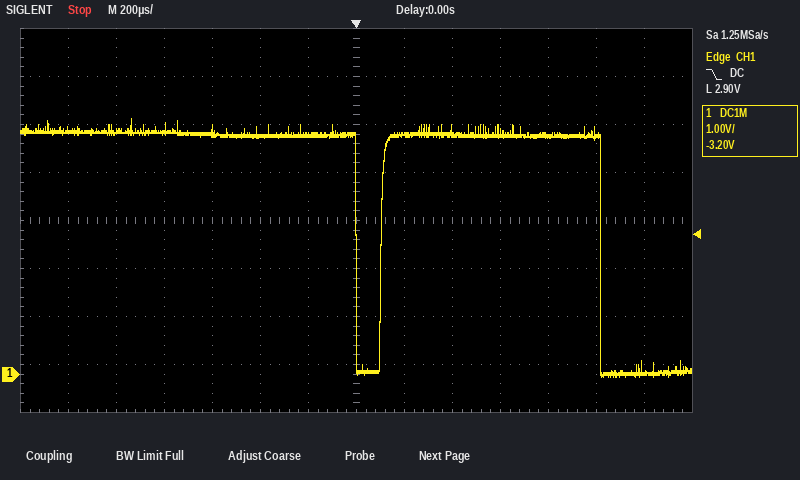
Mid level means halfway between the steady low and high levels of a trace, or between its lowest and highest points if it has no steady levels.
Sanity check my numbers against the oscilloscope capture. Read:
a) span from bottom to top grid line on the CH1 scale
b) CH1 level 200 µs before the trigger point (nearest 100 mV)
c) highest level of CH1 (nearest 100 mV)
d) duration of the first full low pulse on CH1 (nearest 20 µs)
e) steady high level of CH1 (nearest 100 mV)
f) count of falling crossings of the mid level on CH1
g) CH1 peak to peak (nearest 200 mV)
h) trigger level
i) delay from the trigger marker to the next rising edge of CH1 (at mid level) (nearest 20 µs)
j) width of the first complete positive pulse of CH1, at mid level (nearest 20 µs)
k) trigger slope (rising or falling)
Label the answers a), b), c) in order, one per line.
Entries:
a) 8 V
b) 5.0 V
c) 5.3 V
d) 100 µs
e) 5.0 V
f) 2
g) 5.4 V
h) 2.90 V
i) 100 µs
j) 920 µs
k) falling
